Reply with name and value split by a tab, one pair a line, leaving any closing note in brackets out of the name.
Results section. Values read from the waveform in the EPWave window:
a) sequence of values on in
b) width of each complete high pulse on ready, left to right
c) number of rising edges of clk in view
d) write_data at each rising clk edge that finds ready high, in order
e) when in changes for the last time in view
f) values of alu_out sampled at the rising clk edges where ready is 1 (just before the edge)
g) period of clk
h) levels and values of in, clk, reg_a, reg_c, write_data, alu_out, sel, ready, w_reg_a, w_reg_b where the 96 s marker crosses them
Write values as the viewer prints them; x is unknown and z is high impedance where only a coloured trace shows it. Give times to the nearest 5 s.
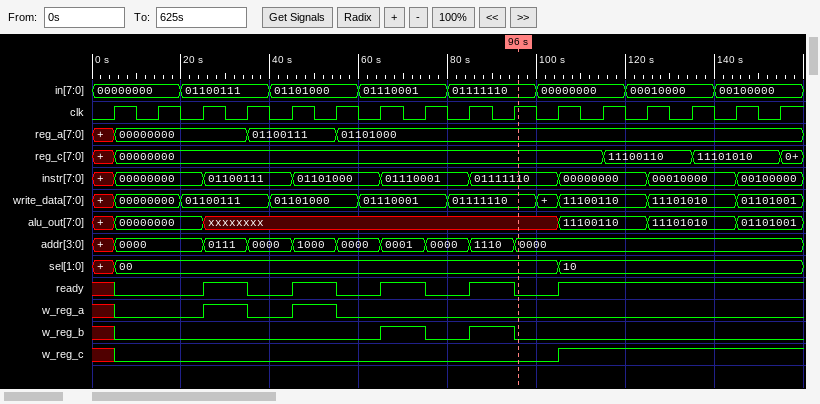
sequence of values on in	00000000, 01100111, 01101000, 01110001, 01111110, 00000000, 00010000, 00100000
width of each complete high pulse on ready, left to right	10 s, 10 s, 10 s, 10 s
number of rising edges of clk in view	16
write_data at each rising clk edge that finds ready high, in order	01100111, 01101000, 01110001, 01111110, 11100110, 11100110, 11101010, 11101010, 01101001
when in changes for the last time in view	140 s
values of alu_out sampled at the rising clk edges where ready is 1	xxxxxxxx, xxxxxxxx, xxxxxxxx, xxxxxxxx, 11100110, 11100110, 11101010, 11101010, 01101001
period of clk	10 s
levels and values of in, clk, reg_a, reg_c, write_data, alu_out, sel, ready, w_reg_a, w_reg_b where the 96 s marker crosses them	in=01111110, clk=1, reg_a=01101000, reg_c=00000000, write_data=01111110, alu_out=xxxxxxxx, sel=00, ready=0, w_reg_a=0, w_reg_b=0
